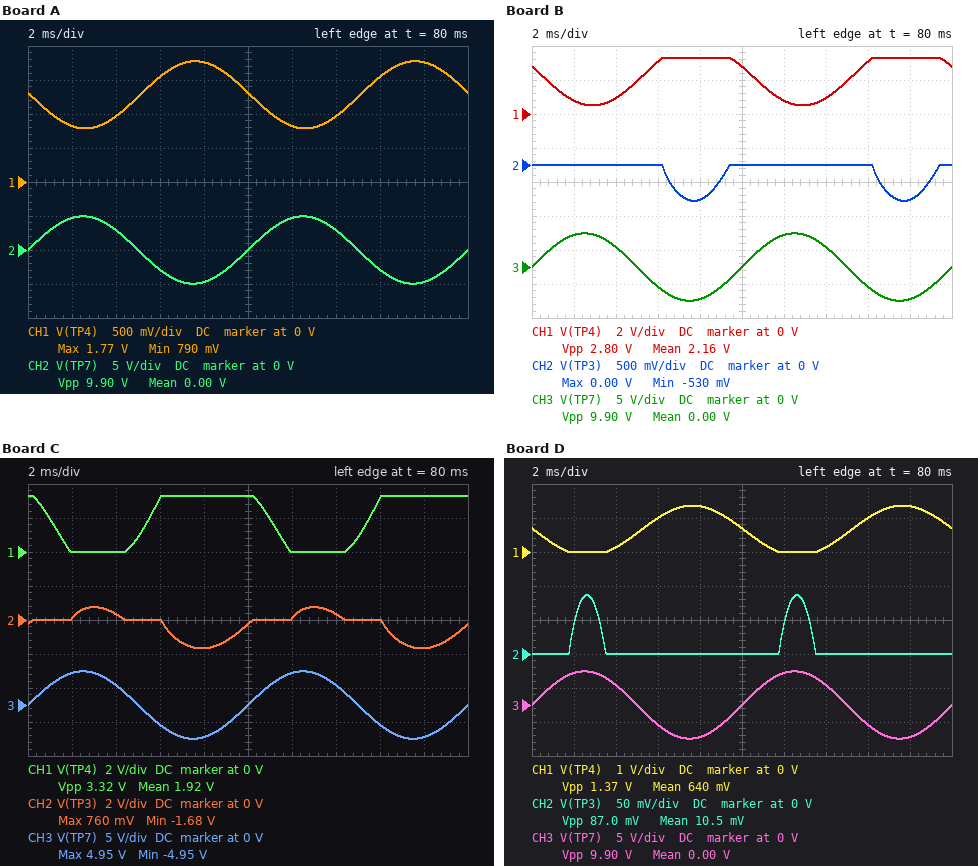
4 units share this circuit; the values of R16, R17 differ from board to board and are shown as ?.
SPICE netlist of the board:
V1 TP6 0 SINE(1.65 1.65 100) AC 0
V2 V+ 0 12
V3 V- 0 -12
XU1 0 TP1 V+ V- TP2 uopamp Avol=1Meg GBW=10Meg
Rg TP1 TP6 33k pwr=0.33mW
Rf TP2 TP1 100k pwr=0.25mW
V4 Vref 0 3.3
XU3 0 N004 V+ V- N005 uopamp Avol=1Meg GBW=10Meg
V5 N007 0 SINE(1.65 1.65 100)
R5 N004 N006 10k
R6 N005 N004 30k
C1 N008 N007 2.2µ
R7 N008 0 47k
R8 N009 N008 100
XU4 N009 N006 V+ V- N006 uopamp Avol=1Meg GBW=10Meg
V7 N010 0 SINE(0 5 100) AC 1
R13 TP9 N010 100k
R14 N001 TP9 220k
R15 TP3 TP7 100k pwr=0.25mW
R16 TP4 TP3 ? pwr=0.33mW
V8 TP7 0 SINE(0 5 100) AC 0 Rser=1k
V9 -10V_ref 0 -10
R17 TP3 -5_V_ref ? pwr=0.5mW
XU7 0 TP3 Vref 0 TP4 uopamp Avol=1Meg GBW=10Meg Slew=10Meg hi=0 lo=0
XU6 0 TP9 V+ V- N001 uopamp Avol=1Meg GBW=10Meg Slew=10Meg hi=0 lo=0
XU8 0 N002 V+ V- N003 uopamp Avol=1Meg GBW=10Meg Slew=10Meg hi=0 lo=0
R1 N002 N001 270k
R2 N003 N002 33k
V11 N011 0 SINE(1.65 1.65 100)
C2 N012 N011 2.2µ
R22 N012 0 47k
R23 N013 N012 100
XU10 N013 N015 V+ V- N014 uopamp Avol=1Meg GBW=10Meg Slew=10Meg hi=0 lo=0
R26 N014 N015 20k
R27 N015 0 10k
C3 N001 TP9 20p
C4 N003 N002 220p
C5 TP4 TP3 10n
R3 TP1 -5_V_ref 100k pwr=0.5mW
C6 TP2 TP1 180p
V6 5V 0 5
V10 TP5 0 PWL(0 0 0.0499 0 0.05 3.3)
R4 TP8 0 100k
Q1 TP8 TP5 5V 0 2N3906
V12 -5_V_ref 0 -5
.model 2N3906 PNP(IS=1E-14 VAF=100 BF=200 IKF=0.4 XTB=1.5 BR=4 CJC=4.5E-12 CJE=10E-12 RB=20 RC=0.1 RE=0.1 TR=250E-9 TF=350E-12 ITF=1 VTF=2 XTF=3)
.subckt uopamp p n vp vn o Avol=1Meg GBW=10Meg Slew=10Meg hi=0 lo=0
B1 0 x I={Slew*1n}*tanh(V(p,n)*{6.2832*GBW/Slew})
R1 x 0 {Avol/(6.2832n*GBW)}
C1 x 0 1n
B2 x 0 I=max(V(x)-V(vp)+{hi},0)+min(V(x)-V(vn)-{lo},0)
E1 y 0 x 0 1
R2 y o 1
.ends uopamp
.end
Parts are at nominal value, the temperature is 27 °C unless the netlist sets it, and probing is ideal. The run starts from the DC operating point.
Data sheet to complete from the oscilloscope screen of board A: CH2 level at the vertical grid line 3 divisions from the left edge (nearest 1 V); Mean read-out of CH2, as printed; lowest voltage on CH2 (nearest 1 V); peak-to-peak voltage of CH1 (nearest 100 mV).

-3 V
0.00 V
-5 V
1.0 V
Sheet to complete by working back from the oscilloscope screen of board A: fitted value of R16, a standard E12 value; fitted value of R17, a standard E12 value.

10 kΩ
39 kΩ
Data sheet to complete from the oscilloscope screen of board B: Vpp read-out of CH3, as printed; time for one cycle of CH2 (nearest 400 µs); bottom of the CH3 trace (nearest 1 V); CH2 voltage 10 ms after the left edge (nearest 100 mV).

9.90 V
10.0 ms
-5 V
0 V
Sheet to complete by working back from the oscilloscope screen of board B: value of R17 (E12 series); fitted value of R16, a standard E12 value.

82 kΩ
39 kΩ
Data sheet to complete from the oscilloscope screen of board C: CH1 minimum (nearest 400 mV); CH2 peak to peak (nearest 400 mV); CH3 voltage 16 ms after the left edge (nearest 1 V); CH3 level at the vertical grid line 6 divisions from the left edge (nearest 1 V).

0 V
2.4 V
-3 V
5 V
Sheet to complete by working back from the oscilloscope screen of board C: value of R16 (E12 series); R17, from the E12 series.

100 kΩ
180 kΩ
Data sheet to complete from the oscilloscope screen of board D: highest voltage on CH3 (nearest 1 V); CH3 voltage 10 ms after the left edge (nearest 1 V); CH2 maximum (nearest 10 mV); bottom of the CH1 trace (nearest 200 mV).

5 V
0 V
90 mV
0 V
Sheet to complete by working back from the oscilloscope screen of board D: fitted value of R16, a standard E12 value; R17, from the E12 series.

15 kΩ
120 kΩ
